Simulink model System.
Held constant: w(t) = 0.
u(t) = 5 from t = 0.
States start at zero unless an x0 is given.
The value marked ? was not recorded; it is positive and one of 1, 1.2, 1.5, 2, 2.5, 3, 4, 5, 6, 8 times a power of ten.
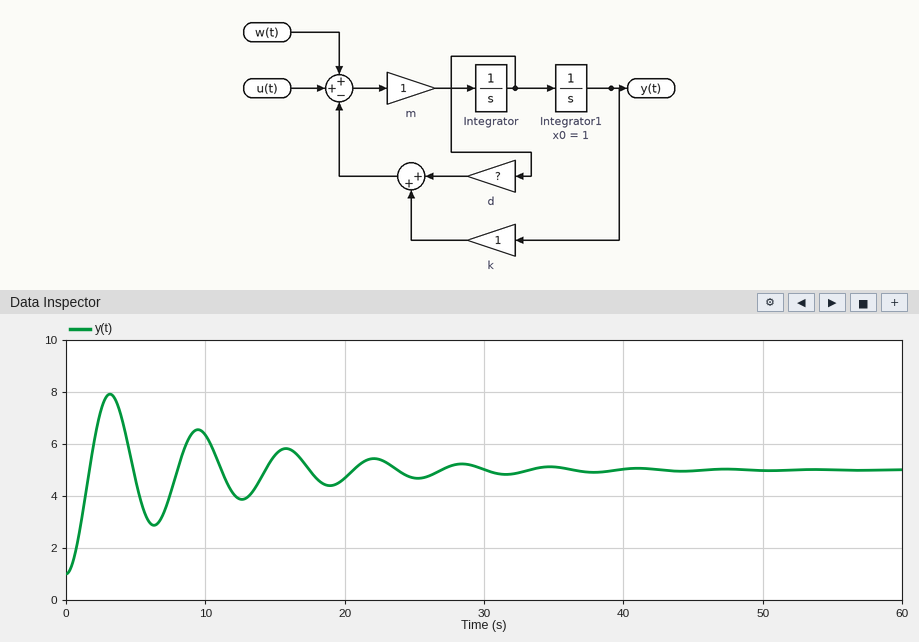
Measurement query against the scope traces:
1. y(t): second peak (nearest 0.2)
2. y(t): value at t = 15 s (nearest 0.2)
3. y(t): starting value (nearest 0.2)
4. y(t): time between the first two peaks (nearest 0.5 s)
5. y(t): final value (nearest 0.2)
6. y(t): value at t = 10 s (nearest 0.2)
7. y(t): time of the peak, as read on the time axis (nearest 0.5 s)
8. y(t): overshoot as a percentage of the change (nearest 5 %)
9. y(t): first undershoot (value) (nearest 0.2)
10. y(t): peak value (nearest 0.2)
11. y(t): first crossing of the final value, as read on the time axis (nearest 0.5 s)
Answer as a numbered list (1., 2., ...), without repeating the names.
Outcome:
1. 6.6
2. 5.6
3. 1.0
4. 6.5 s
5. 5.0
6. 6.4
7. 3.0 s
8. 75 %
9. 2.8
10. 8.0
11. 1.5 s
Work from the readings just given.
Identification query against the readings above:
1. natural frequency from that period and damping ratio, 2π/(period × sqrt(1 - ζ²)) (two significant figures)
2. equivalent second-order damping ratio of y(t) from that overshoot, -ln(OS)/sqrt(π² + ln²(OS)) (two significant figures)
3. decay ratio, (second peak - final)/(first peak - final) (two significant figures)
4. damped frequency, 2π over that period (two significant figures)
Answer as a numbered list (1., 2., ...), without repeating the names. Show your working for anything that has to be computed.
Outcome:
1. 2π / (6.5 × sqrt(1 - 0.091²)) = 0.97 rad/s
2. ln(0.75) = -0.288; 0.288 / sqrt(9.870 + 0.083) = 0.091
3. (6.6 - 5) / (8 - 5) = 0.53
4. 2π / 6.5 = 0.97 rad/s
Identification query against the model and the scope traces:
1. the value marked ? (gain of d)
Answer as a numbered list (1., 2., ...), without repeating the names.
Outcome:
1. 0.2
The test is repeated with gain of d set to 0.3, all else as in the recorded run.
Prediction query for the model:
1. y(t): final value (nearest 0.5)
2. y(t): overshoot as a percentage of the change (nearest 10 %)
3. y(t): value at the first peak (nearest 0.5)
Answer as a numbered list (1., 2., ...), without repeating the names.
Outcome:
1. 5.0
2. 60 %
3. 7.5
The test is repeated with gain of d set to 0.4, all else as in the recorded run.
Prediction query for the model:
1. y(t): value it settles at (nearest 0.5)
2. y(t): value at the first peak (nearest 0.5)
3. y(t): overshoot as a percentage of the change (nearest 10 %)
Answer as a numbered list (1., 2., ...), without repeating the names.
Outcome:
1. 5.0
2. 7.0
3. 50 %
